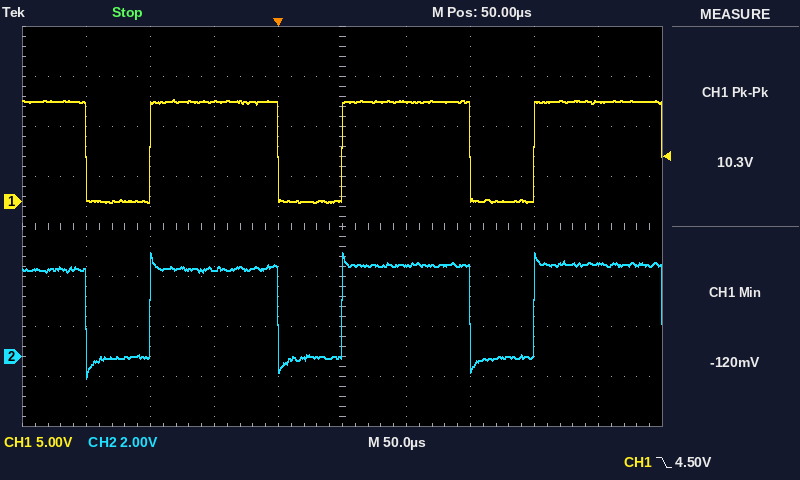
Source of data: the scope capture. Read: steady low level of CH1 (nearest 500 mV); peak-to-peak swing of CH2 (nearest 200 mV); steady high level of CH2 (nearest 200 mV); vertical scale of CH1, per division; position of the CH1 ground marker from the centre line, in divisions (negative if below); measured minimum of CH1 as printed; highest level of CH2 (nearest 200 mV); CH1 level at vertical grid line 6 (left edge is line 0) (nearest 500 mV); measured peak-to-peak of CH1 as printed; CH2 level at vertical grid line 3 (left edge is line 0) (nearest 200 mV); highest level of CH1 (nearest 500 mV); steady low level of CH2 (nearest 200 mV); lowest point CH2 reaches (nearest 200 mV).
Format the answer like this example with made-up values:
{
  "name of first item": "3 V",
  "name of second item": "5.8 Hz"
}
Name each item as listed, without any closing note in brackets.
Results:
{
  "steady low level of CH1": "0.0 V",
  "peak-to-peak swing of CH2": "5.0 V",
  "steady high level of CH2": "3.6 V",
  "vertical scale of CH1, per division": "5 V",
  "position of the CH1 ground marker from the centre line, in divisions": "+0.5 div",
  "measured minimum of CH1 as printed": "-120 mV",
  "highest level of CH2": "4.2 V",
  "CH1 level at vertical grid line 6 (left edge is line 0)": "10.0 V",
  "measured peak-to-peak of CH1 as printed": "10.3 V",
  "CH2 level at vertical grid line 3 (left edge is line 0)": "3.4 V",
  "highest level of CH1": "10.0 V",
  "steady low level of CH2": "0.0 V",
  "lowest point CH2 reaches": "-800 mV"
}
